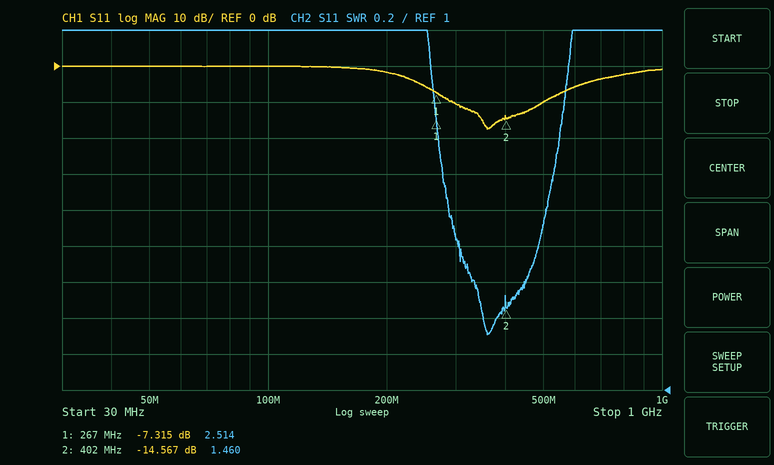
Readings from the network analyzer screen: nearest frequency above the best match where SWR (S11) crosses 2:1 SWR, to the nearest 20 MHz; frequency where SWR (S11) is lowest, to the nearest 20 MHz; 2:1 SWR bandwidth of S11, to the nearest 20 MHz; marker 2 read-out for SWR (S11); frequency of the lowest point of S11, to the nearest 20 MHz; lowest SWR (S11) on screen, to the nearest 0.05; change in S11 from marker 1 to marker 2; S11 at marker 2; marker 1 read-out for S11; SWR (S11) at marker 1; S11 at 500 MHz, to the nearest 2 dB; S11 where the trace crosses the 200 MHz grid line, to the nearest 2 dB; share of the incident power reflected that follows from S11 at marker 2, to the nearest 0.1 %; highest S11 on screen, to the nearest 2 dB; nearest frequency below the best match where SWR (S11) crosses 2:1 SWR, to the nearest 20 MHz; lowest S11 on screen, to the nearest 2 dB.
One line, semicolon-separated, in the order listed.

500 MHz; 360 MHz; 220 MHz; 1.460; 360 MHz; 1.30; -7.252 dB; -14.567 dB; -7.315 dB; 2.514; -10 dB; -2 dB; 3.5 %; 0 dB; 280 MHz; -18 dB
